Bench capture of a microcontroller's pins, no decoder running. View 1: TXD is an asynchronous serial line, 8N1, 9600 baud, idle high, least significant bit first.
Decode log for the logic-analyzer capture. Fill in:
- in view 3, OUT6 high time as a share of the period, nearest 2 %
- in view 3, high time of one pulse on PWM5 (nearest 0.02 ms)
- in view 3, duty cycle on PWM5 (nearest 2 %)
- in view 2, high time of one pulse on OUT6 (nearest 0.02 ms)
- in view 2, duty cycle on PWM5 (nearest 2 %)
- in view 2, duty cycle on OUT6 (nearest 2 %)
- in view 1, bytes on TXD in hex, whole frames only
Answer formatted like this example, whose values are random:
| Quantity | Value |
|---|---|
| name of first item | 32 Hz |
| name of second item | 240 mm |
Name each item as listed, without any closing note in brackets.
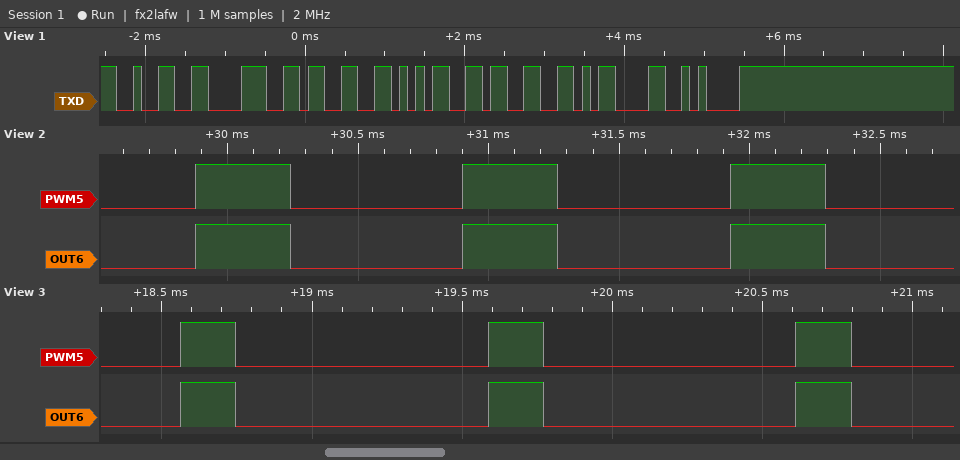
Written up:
| Quantity | Value |
|---|---|
| in view 3, OUT6 high time as a share of the period, nearest 2 % | 18 % |
| in view 3, high time of one pulse on PWM5 | 0.18 ms |
| in view 3, duty cycle on PWM5 | 18 % |
| in view 2, high time of one pulse on OUT6 | 0.36 ms |
| in view 2, duty cycle on PWM5 | 36 % |
| in view 2, duty cycle on OUT6 | 36 % |
| in view 1, bytes on TXD in hex, whole frames only | 32 38 33 35 33 0D 0A |
